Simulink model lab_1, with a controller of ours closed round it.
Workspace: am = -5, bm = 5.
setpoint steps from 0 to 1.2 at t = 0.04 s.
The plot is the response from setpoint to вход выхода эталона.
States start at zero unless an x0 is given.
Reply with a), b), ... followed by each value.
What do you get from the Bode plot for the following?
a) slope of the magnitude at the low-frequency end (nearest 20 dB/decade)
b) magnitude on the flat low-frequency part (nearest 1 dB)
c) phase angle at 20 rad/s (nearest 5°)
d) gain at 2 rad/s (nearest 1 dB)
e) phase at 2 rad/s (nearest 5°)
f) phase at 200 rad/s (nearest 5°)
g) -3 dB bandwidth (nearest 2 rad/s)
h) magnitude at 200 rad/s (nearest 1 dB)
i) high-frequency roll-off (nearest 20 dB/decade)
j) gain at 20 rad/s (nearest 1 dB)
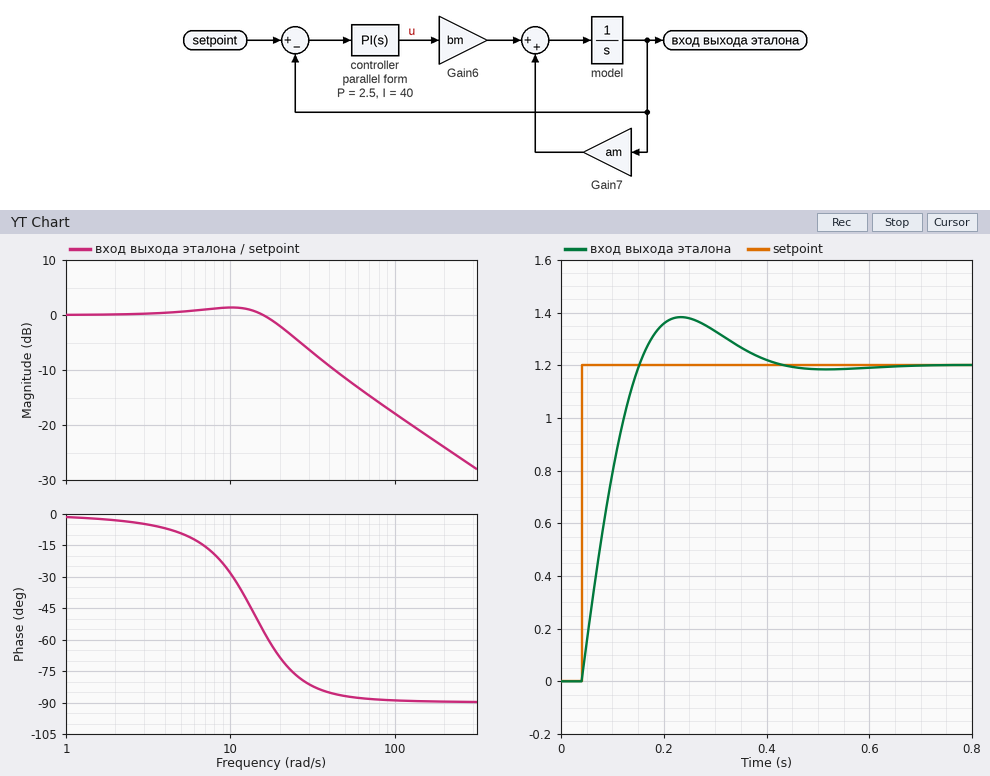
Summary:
a) 0 dB/decade
b) 0 dB
c) -70°
d) 0 dB
e) -5°
f) -90°
g) 22 rad/s
h) -24 dB
i) -20 dB/decade
j) -2 dB
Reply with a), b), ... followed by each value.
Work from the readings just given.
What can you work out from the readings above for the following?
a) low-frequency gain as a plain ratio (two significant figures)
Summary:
a) 1.0
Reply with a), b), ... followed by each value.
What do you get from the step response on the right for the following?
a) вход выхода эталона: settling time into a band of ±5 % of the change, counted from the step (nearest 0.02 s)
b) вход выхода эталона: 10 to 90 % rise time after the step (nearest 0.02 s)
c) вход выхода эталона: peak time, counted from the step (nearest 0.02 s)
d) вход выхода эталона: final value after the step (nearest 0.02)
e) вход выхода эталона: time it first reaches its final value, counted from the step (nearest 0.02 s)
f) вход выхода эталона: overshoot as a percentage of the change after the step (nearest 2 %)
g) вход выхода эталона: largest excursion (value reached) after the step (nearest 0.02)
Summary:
a) 0.32 s
b) 0.08 s
c) 0.20 s
d) 1.20
e) 0.12 s
f) 16 %
g) 1.38
